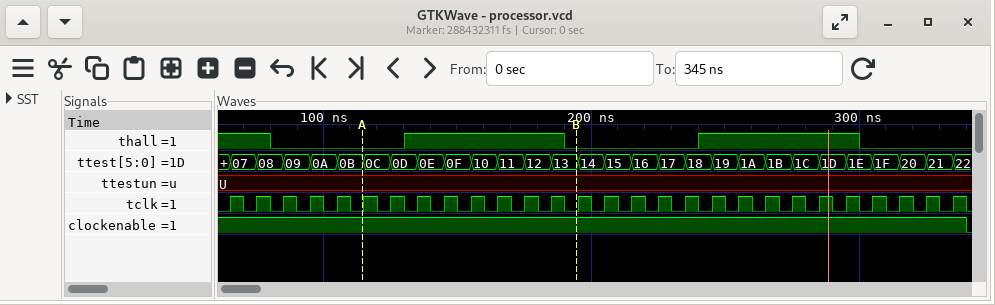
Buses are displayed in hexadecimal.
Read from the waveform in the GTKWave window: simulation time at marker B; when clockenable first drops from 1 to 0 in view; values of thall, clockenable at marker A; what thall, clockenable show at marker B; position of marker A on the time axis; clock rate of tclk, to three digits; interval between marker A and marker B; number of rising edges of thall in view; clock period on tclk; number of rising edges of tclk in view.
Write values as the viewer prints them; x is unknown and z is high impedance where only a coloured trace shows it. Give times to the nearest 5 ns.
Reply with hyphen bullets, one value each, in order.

- 195 ns
- 340 ns
- thall=0, clockenable=1
- thall=0, clockenable=1
- 115 ns
- 100 MHz
- 80 ns
- 2
- 10 ns
- 28
